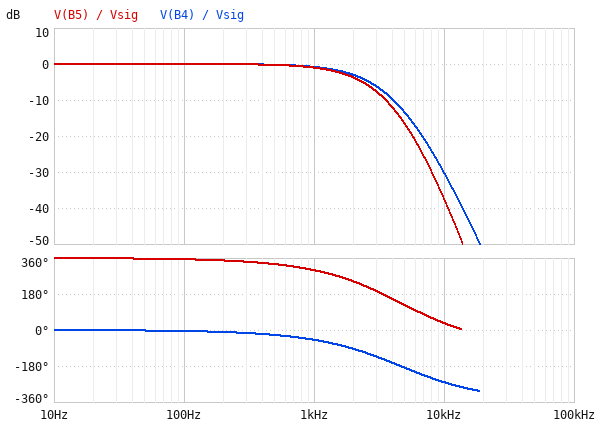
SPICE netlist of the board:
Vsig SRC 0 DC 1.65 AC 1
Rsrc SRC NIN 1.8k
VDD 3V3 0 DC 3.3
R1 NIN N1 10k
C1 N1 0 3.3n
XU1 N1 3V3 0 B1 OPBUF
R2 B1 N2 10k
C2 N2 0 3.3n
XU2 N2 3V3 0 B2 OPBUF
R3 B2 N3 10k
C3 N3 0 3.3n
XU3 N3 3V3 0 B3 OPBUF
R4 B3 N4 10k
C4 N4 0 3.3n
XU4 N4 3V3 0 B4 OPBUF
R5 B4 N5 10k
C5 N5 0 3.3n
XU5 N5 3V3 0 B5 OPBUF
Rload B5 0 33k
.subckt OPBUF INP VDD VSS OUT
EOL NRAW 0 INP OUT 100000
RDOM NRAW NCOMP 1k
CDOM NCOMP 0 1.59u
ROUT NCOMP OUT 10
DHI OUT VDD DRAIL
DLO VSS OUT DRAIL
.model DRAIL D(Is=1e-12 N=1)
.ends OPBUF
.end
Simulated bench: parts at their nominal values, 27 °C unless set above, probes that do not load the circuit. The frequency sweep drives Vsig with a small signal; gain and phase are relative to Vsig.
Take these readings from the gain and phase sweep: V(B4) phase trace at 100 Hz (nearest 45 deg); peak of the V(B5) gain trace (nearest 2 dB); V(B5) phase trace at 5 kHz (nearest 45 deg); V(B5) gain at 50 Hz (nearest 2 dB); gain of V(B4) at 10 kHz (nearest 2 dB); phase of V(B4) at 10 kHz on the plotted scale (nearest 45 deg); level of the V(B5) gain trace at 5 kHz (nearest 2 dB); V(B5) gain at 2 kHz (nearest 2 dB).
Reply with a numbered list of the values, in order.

1. 0 deg
2. 0 dB
3. 135 deg
4. 0 dB
5. -30 dB
6. -270 deg
7. -16 dB
8. -4 dB
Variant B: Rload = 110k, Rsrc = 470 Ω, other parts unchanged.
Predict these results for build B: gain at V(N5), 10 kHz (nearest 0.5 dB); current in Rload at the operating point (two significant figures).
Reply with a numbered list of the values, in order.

1. -36.5 dB
2. 15 µA
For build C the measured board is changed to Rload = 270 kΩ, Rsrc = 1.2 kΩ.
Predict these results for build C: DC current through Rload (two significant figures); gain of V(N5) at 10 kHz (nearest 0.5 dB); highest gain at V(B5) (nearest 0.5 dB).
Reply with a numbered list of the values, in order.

1. 6.1 µA
2. -37.0 dB
3. 0 dB
